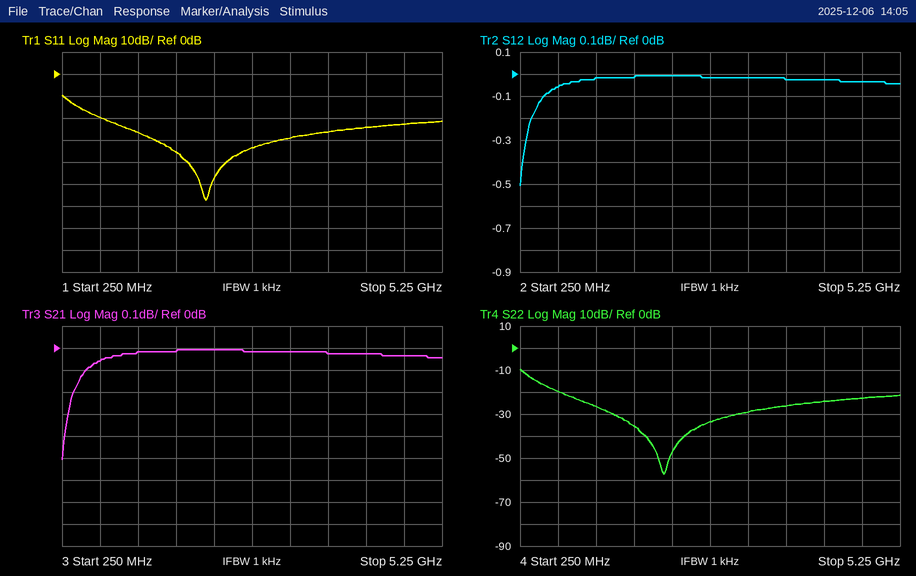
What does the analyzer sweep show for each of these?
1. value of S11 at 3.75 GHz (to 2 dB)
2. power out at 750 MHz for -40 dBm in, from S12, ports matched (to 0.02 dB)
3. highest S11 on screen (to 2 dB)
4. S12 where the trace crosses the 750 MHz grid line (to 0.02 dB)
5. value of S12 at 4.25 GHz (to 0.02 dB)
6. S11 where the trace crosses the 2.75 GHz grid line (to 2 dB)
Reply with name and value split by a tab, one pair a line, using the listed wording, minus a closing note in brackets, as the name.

value of S11 at 3.75 GHz	-26 dB
power out at 750 MHz for -40 dBm in, from S12, ports matched	-40.06 dBm
highest S11 on screen	-10 dB
S12 where the trace crosses the 750 MHz grid line	-0.06 dB
value of S12 at 4.25 GHz	-0.02 dB
S11 where the trace crosses the 2.75 GHz grid line	-34 dB
